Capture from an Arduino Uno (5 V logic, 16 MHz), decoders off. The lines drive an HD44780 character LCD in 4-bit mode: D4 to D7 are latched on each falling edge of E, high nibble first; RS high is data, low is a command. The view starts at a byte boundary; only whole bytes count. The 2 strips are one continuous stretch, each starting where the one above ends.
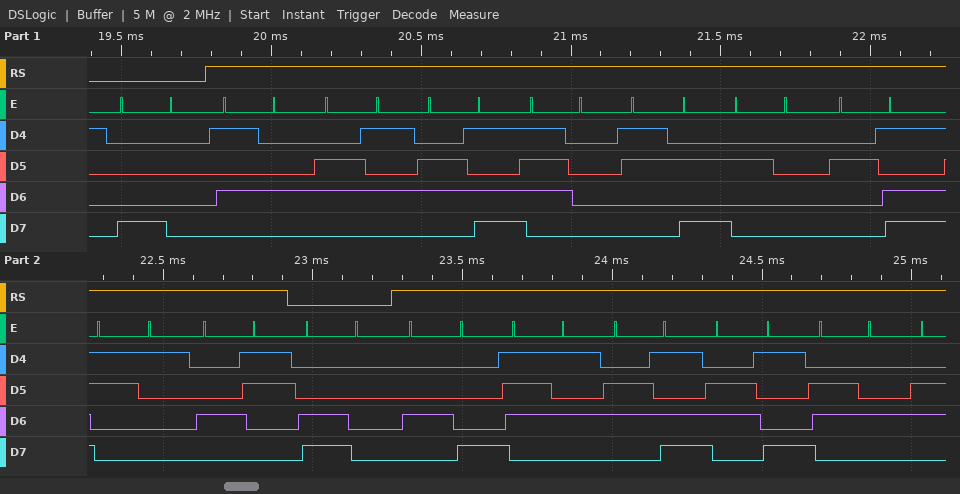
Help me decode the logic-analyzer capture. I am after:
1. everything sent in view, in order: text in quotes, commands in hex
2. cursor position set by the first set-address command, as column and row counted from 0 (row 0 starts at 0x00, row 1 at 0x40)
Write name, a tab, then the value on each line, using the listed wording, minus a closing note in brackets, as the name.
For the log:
everything sent in view, in order: text in quotes, commands in hex	0x80 "Temp: -1C" 0xC0 "Humid"
cursor position set by the first set-address command, as column and row counted from 0	column 0, row 0
